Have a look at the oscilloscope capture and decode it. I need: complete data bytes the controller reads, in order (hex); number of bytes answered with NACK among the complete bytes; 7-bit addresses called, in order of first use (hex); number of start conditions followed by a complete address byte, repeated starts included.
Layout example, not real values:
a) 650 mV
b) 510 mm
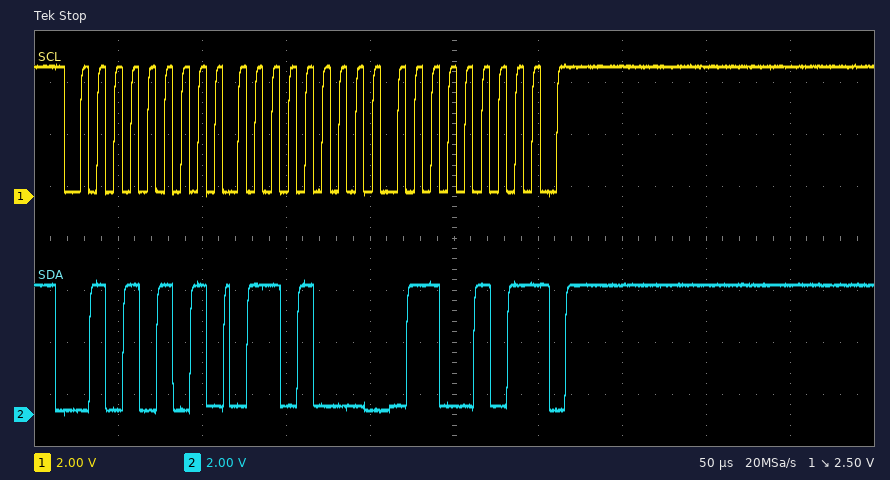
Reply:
a) 68 65
b) 1
c) 0x2A
d) 1
